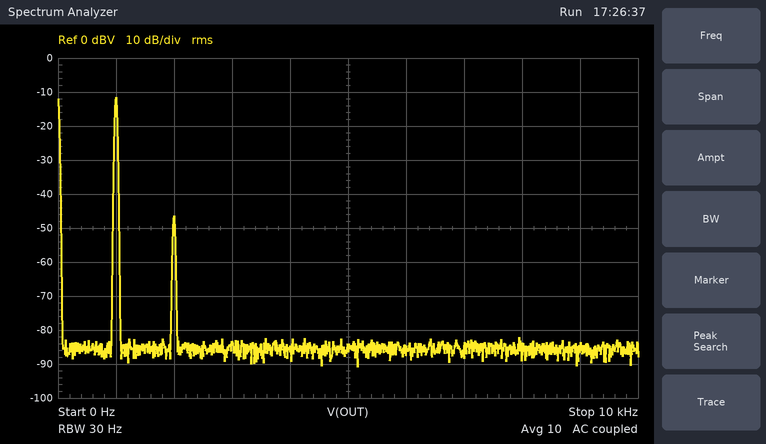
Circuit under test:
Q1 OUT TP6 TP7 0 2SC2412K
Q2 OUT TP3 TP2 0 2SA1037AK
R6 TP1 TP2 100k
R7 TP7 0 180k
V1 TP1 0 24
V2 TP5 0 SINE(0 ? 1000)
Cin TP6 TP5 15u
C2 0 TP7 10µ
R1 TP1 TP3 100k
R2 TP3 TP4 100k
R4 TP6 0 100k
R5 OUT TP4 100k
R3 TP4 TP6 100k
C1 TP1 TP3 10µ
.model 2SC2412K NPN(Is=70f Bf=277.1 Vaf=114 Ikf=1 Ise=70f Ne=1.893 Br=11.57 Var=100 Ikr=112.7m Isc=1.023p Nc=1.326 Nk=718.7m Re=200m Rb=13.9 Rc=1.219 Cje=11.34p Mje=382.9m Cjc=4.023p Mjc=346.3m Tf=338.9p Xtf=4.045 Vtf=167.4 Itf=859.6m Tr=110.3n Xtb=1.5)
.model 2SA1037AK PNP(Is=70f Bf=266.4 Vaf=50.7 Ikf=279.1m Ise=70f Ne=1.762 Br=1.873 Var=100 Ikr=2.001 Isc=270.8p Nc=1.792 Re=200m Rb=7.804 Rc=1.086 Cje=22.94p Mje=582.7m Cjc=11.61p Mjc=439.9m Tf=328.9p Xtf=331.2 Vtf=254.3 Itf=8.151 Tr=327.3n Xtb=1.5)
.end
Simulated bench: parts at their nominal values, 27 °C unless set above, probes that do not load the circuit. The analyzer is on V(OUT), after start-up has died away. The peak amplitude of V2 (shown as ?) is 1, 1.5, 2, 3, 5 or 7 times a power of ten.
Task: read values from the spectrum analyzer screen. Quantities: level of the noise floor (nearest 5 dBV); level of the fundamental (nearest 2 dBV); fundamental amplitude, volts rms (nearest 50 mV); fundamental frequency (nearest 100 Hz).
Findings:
-85 dBV
-12 dBV
250 mV
1.0 kHz
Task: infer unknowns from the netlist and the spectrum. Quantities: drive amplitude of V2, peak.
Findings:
2 mV
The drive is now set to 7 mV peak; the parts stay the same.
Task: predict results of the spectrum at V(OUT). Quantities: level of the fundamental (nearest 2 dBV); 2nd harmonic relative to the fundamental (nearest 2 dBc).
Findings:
0 dBV
-24 dBc
